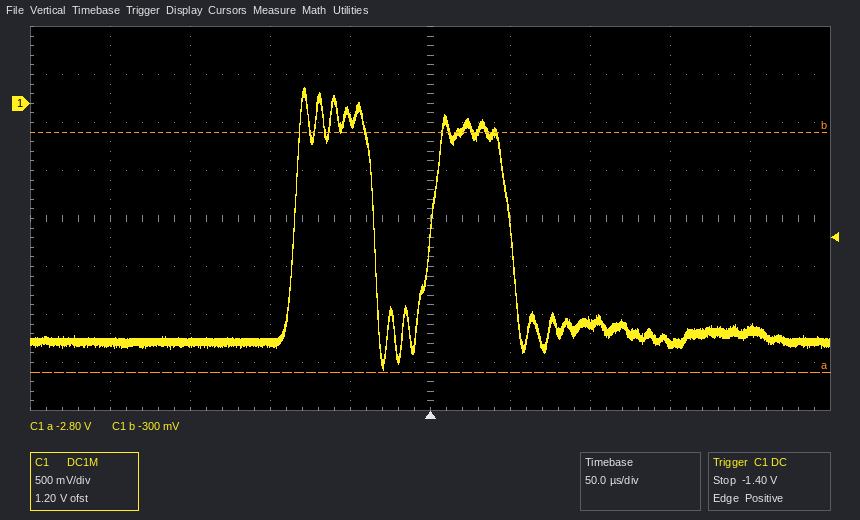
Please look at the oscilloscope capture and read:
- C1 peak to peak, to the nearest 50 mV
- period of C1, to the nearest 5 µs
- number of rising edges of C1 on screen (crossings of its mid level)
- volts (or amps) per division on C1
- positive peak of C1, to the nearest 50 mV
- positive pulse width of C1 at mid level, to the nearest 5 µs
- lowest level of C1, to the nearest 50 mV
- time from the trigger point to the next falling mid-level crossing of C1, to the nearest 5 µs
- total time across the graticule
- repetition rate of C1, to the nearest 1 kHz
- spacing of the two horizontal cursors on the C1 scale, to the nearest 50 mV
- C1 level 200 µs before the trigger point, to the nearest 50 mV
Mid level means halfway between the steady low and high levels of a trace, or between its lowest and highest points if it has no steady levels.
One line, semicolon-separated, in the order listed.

2.95 V; 85 µs; 2; 500 mV; 150 mV; 50 µs; -2.80 V; 50 µs; 500 µs; 12 kHz; 2.50 V; -2.50 V
